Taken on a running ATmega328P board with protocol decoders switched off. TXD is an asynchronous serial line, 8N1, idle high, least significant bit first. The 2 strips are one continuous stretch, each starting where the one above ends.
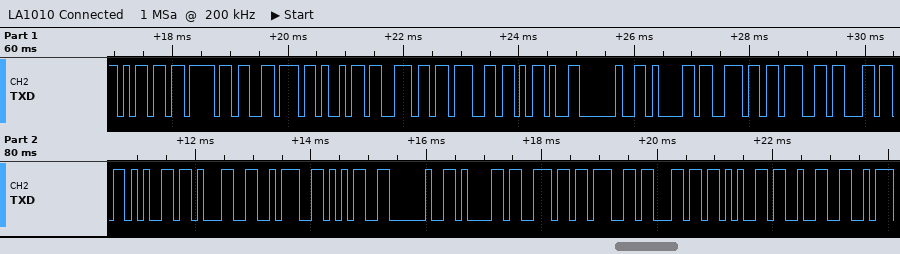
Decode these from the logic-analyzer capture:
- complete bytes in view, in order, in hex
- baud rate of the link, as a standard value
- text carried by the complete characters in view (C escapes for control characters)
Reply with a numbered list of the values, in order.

1. 6D 6F 76 69 6E 67 2D 20 61 6E 67 6C 65 31 3A 35 20 61 6E 67 6C 65 32
2. 9600 baud
3. "moving- angle1:5 angle2"
